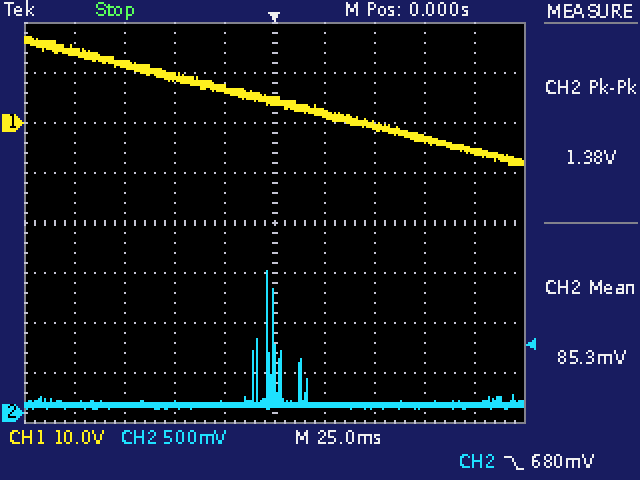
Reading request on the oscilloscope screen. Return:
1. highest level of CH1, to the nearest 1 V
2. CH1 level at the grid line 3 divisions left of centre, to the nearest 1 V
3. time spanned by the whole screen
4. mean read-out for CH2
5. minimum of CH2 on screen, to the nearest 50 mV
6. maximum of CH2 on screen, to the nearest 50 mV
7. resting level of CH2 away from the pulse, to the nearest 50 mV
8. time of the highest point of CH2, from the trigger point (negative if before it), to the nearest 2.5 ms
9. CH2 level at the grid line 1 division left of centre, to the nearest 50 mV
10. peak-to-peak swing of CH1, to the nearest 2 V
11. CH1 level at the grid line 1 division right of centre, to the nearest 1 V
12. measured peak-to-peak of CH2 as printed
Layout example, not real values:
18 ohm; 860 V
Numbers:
17 V; 12 V; 250 ms; 85.3 mV; 50 mV; 1.40 V; 100 mV; -2.5 ms; 100 mV; 26 V; 2 V; 1.38 V
